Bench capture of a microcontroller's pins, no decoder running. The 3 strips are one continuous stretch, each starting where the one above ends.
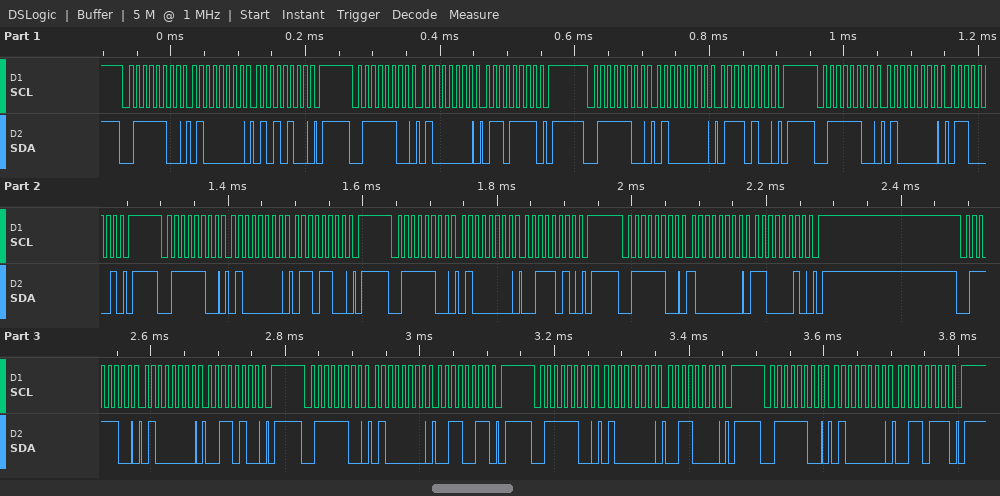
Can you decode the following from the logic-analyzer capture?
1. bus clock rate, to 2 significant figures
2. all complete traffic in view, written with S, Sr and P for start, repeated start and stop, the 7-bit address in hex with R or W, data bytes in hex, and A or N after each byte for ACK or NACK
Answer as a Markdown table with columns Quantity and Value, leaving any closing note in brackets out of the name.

| Quantity | Value |
|---|---|
| bus clock rate, to 2 significant figures | 100 kHz |
| all complete traffic in view, written with S, Sr and P for start, repeated start and stop, the 7-bit address in hex with R or W, data bytes in hex, and A or N after each byte for ACK or NACK | S 3EW A 40 A 54 A P S 3EW A 40 A 6F A P S 3EW A 40 A 74 A P S 3EW A 40 A 61 A P S 3EW A 40 A 6C A P S 3EW A 40 A 3A A P S 3EW A 80 A C2 A P S 3EW A 40 A 34 A P S 3EW A 40 A 33 A P S 3EW A 40 A 30 A P S 3EW A 40 A 37 A P |
